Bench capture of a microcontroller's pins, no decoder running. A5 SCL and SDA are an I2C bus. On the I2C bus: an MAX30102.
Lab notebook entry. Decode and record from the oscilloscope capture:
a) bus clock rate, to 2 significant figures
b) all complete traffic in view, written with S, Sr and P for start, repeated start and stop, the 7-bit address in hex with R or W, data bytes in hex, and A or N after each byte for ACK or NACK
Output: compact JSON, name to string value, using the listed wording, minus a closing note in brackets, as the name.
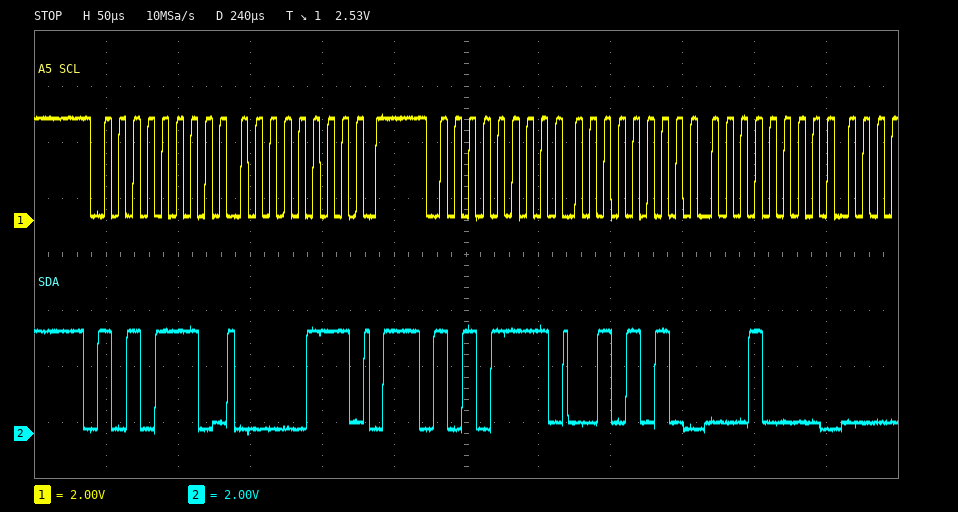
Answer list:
{"bus clock rate, to 2 significant figures": "100 kHz", "all complete traffic in view, written with S, Sr and P for start, repeated start and stop, the 7-bit address in hex with R or W, data bytes in hex, and A or N after each byte for ACK or NACK": "S 57W A 07 A P S 57R A 2A A 10 A"}
